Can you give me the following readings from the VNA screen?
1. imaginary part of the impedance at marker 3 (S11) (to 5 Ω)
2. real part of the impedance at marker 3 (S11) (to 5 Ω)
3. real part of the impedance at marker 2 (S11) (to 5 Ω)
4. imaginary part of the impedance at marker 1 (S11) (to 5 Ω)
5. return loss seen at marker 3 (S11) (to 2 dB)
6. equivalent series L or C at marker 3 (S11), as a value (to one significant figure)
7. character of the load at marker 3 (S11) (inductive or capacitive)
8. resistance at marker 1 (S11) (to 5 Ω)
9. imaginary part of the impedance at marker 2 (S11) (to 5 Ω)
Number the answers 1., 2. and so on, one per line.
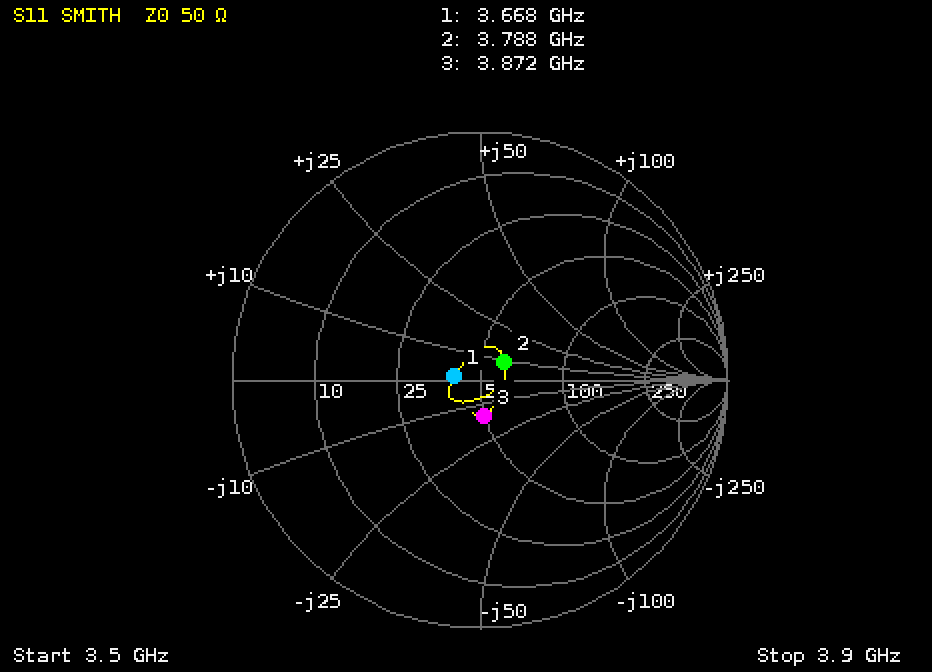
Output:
1. -15 Ω
2. 50 Ω
3. 60 Ω
4. 0 Ω
5. 16 dB
6. 3 pF
7. capacitive
8. 40 Ω
9. +10 Ω
